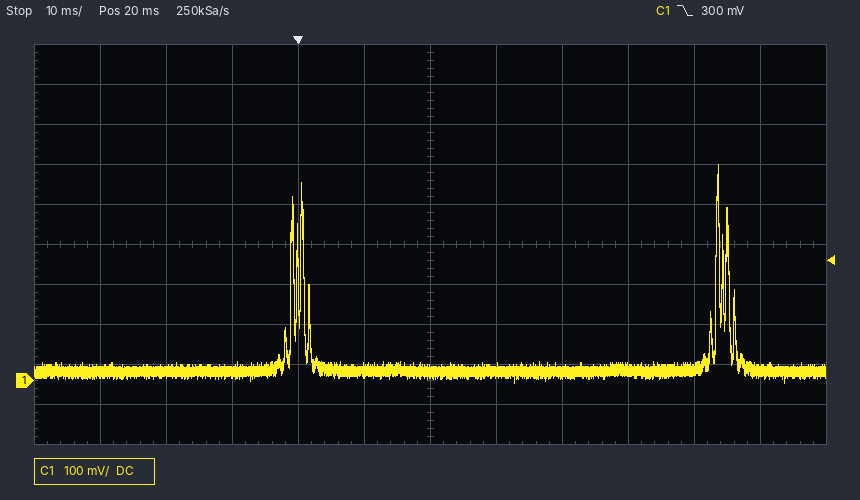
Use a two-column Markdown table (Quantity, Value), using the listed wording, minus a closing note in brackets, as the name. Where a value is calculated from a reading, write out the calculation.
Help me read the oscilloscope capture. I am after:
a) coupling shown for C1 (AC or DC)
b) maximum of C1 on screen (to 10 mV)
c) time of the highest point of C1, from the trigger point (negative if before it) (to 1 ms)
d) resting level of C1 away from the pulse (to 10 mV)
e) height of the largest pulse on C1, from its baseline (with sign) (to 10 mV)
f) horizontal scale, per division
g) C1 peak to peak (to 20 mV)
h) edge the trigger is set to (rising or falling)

| Quantity | Value |
|---|---|
| coupling shown for C1 | DC |
| maximum of C1 on screen | 540 mV |
| time of the highest point of C1, from the trigger point (negative if before it) | +64 ms |
| resting level of C1 away from the pulse | 20 mV |
| height of the largest pulse on C1, from its baseline (with sign) | 540 mV − (20 mV) = +520 mV |
| horizontal scale, per division | 10 ms |
| C1 peak to peak | 540 mV |
| edge the trigger is set to | falling |
